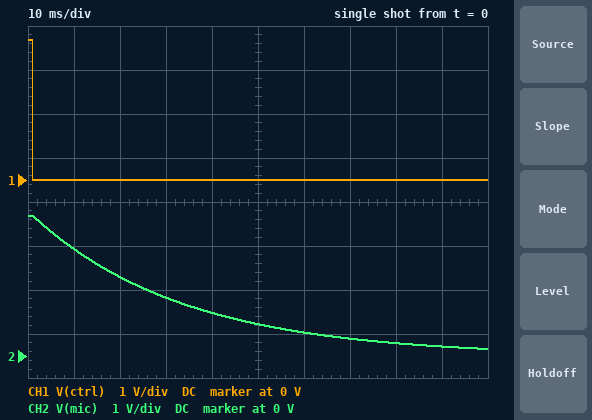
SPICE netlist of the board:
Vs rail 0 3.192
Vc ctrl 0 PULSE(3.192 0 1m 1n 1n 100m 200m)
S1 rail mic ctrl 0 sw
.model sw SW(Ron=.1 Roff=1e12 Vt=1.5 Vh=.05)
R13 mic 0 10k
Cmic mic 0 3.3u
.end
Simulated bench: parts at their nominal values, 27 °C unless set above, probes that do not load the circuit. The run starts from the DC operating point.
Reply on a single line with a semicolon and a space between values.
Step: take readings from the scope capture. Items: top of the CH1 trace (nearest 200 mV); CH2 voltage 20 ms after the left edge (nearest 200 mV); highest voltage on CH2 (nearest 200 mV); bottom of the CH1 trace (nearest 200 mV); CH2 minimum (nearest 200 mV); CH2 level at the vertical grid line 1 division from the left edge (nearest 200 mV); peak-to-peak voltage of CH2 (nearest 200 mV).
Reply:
3.2 V; 1.8 V; 3.2 V; 0 V; 200 mV; 2.4 V; 3.0 V
